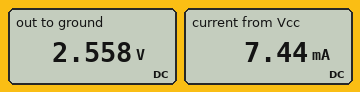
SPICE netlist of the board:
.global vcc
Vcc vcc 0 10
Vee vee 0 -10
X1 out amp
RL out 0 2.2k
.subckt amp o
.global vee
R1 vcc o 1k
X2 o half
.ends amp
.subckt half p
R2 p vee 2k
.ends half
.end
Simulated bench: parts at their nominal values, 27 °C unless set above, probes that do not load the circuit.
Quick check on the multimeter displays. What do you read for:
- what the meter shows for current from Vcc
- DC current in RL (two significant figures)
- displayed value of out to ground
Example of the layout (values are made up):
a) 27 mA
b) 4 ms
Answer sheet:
a) 7.44 mA
b) 1.2 mA
c) 2.558 V
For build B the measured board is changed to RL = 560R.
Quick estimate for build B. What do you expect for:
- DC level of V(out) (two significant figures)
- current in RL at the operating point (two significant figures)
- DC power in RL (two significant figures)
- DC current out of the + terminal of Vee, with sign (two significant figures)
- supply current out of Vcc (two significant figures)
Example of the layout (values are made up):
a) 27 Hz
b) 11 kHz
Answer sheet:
a) 1.5 V
b) 2.7 mA
c) 4.1 mW
d) -5.8 mA
e) 8.5 mA
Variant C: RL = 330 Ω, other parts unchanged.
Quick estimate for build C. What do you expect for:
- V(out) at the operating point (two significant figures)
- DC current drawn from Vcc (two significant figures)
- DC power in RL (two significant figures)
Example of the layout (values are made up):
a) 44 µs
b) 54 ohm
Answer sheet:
a) 1.1 V
b) 8.9 mA
c) 3.7 mW
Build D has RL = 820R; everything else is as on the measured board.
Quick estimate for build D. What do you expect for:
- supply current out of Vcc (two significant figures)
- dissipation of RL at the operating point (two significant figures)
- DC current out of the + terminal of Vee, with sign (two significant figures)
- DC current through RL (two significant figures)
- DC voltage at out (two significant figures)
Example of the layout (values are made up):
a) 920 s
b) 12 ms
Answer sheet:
a) 8.2 mA
b) 4.1 mW
c) -5.9 mA
d) 2.2 mA
e) 1.8 V
